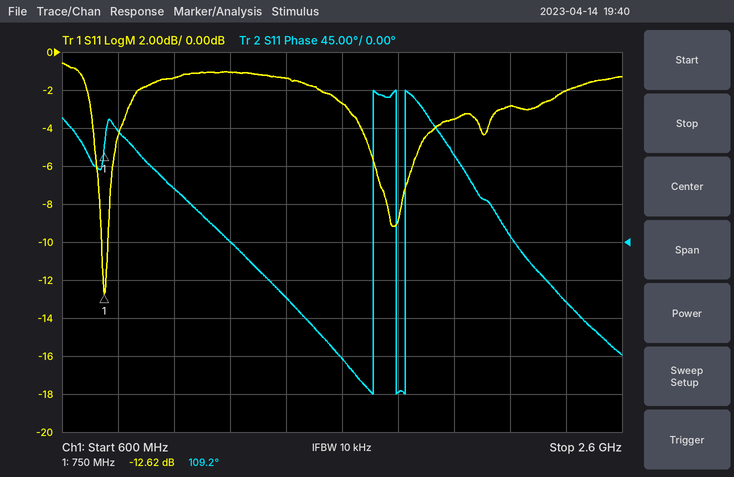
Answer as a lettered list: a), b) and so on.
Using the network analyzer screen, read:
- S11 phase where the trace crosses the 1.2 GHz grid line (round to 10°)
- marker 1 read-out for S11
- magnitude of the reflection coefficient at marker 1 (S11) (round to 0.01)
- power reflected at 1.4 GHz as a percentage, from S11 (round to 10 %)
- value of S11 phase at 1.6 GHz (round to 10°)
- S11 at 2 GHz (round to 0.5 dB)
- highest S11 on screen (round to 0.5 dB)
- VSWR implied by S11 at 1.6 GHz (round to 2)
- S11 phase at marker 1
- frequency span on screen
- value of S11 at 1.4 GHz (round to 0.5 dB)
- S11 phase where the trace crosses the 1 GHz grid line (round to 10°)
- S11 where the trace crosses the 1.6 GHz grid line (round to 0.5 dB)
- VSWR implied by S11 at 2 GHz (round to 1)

a) 0°
b) -12.62 dB
c) 0.23
d) 70 %
e) -140°
f) -3.5 dB
g) -0.5 dB
h) 6
i) 109.2°
j) 2 GHz
k) -1.5 dB
l) 60°
m) -2.5 dB
n) 5
